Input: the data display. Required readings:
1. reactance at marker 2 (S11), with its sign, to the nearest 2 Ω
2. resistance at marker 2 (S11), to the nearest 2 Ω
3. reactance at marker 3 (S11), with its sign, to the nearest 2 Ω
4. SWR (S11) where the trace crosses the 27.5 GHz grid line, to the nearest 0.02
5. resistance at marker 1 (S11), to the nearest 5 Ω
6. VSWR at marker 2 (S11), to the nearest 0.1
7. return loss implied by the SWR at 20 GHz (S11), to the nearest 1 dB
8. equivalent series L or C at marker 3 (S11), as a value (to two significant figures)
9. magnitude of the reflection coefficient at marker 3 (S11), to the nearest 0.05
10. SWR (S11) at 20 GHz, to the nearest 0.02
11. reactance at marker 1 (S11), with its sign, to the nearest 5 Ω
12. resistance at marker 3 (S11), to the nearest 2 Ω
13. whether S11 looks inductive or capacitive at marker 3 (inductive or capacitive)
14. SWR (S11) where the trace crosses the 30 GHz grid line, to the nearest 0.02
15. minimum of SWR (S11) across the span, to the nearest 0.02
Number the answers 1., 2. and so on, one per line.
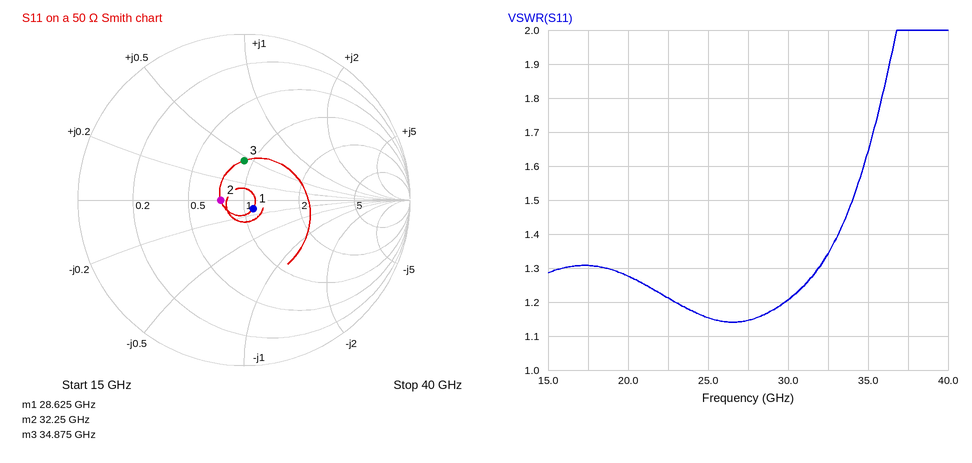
1. 0 Ω
2. 38 Ω
3. +22 Ω
4. 1.14
5. 55 Ω
6. 1.3
7. 18 dB
8. 100 pH
9. 0.25
10. 1.28
11. -5 Ω
12. 44 Ω
13. inductive
14. 1.20
15. 1.14
